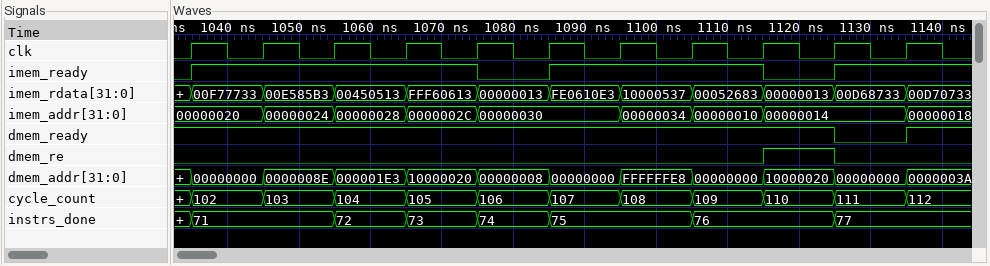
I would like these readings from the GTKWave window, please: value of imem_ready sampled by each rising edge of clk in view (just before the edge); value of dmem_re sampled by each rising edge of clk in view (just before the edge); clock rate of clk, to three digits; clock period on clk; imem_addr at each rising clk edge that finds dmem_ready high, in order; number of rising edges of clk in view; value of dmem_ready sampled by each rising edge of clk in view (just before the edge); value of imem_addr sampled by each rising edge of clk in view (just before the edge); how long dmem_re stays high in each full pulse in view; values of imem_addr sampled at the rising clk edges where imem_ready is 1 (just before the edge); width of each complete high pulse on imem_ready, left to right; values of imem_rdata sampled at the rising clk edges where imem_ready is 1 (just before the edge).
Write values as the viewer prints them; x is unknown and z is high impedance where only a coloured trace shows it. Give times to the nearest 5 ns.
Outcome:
0 1 1 1 1 0 1 1 1 0 1
0 0 0 0 0 0 0 0 0 1 0
100 MHz
10 ns
00000020, 00000020, 00000024, 00000028, 0000002C, 00000030, 00000030, 00000034, 00000010, 00000014
11
1 1 1 1 1 1 1 1 1 1 0
00000020, 00000020, 00000024, 00000028, 0000002C, 00000030, 00000030, 00000034, 00000010, 00000014, 00000014
10 ns
00000020, 00000024, 00000028, 0000002C, 00000030, 00000034, 00000010, 00000014
40 ns, 30 ns
00F77733, 00E585B3, 00450513, FFF60613, FE0610E3, 10000537, 00052683, 00D68733
